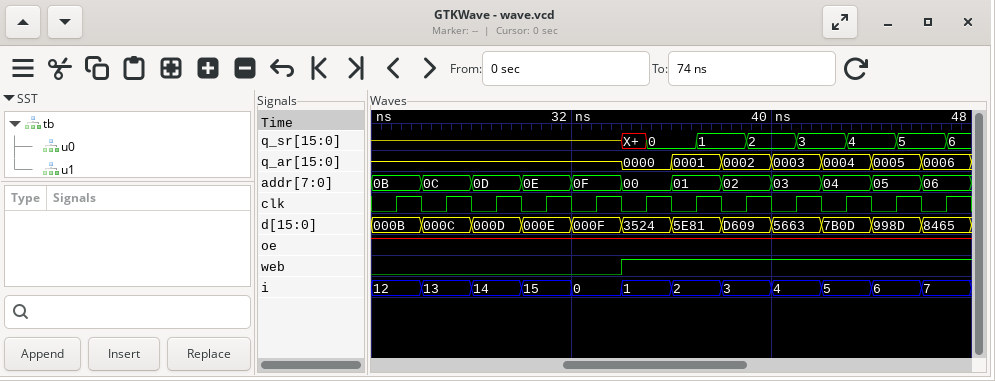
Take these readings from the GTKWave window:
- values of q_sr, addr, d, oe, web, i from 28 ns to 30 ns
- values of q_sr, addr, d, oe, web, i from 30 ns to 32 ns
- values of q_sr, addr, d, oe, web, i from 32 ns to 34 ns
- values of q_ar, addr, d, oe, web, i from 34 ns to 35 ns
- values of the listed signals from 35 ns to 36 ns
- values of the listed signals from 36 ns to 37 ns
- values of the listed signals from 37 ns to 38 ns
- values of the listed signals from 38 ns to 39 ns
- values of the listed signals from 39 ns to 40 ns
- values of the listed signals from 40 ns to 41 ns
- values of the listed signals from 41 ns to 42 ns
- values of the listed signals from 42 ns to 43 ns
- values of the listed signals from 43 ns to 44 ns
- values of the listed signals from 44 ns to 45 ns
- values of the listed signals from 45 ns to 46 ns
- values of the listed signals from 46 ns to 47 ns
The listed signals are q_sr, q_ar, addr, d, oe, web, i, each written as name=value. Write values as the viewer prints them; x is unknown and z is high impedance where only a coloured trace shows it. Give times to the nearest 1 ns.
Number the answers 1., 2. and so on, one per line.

1. q_sr=z, addr=0D, d=000D, oe=1, web=0, i=14
2. q_sr=z, addr=0E, d=000E, oe=1, web=0, i=15
3. q_sr=z, addr=0F, d=000F, oe=1, web=0, i=0
4. q_ar=0000, addr=00, d=3524, oe=1, web=1, i=1
5. q_sr=0, q_ar=0000, addr=00, d=3524, oe=1, web=1, i=1
6. q_sr=0, q_ar=0001, addr=01, d=5E81, oe=1, web=1, i=2
7. q_sr=1, q_ar=0001, addr=01, d=5E81, oe=1, web=1, i=2
8. q_sr=1, q_ar=0002, addr=02, d=D609, oe=1, web=1, i=3
9. q_sr=2, q_ar=0002, addr=02, d=D609, oe=1, web=1, i=3
10. q_sr=2, q_ar=0003, addr=03, d=5663, oe=1, web=1, i=4
11. q_sr=3, q_ar=0003, addr=03, d=5663, oe=1, web=1, i=4
12. q_sr=3, q_ar=0004, addr=04, d=7B0D, oe=1, web=1, i=5
13. q_sr=4, q_ar=0004, addr=04, d=7B0D, oe=1, web=1, i=5
14. q_sr=4, q_ar=0005, addr=05, d=998D, oe=1, web=1, i=6
15. q_sr=5, q_ar=0005, addr=05, d=998D, oe=1, web=1, i=6
16. q_sr=5, q_ar=0006, addr=06, d=8465, oe=1, web=1, i=7
